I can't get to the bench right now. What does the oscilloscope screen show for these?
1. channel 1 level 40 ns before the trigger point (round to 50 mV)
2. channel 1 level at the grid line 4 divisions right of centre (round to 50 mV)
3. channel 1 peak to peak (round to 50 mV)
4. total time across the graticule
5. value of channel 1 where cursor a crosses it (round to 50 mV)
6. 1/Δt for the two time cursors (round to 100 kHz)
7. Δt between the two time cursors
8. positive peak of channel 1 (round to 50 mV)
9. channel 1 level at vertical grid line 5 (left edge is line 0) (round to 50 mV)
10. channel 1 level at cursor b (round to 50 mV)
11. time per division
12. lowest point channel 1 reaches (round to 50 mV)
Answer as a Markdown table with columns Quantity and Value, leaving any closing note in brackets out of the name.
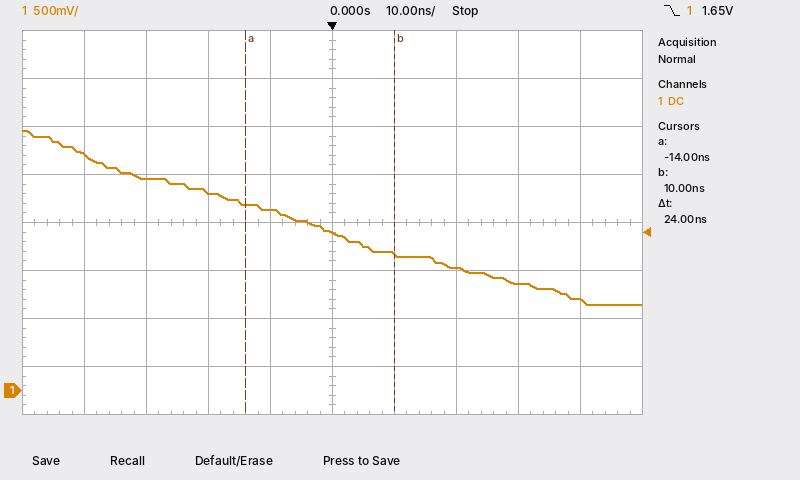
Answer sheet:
| Quantity | Value |
|---|---|
| channel 1 level 40 ns before the trigger point | 2.45 V |
| channel 1 level at the grid line 4 divisions right of centre | 950 mV |
| channel 1 peak to peak | 1.80 V |
| total time across the graticule | 100 ns |
| value of channel 1 where cursor a crosses it | 1.95 V |
| 1/Δt for the two time cursors | 41.7 MHz |
| Δt between the two time cursors | 24 ns |
| positive peak of channel 1 | 2.70 V |
| channel 1 level at vertical grid line 5 (left edge is line 0) | 1.65 V |
| channel 1 level at cursor b | 1.40 V |
| time per division | 10 ns |
| lowest point channel 1 reaches | 900 mV |
